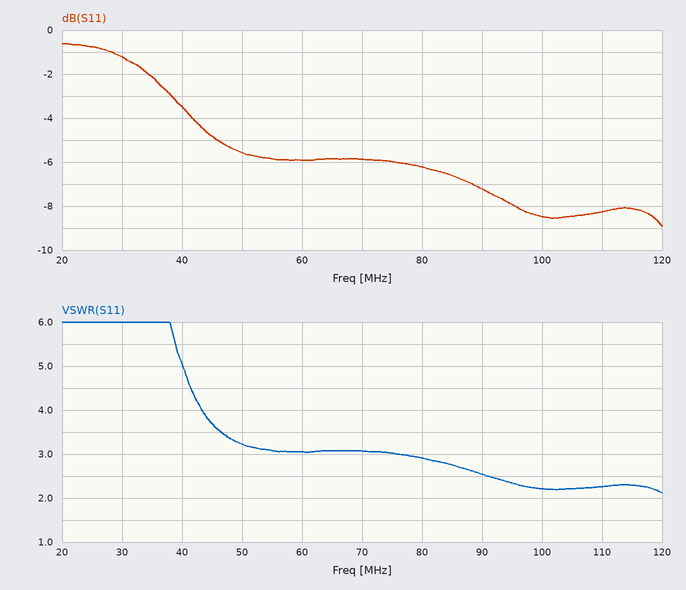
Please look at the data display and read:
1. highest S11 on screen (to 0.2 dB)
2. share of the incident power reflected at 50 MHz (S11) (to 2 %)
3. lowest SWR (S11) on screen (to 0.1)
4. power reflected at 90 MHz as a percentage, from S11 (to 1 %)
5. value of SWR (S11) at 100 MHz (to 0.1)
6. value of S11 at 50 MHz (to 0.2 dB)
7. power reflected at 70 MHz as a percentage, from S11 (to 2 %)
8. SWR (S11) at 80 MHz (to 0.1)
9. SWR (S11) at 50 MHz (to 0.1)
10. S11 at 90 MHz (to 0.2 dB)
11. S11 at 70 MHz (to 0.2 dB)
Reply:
-0.6 dB
28 %
2.1
19 %
2.2
-5.6 dB
26 %
2.9
3.2
-7.2 dB
-5.8 dB
